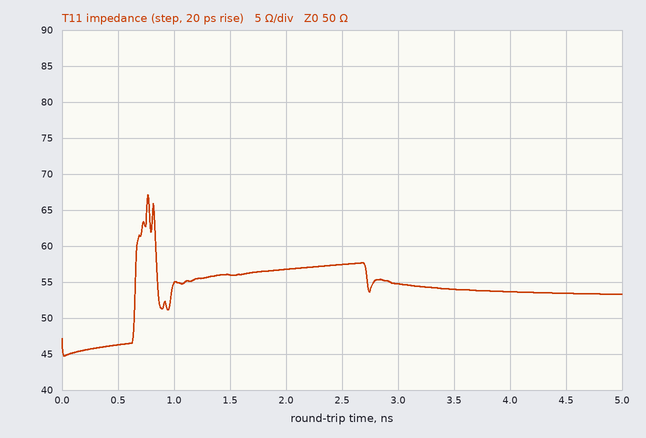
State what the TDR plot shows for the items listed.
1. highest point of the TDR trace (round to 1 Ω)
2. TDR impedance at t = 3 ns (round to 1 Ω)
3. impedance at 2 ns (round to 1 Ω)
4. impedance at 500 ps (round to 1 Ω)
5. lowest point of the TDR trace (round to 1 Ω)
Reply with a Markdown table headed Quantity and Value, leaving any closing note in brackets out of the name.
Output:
| Quantity | Value |
|---|---|
| highest point of the TDR trace | 67 Ω |
| TDR impedance at t = 3 ns | 55 Ω |
| impedance at 2 ns | 57 Ω |
| impedance at 500 ps | 46 Ω |
| lowest point of the TDR trace | 45 Ω |
